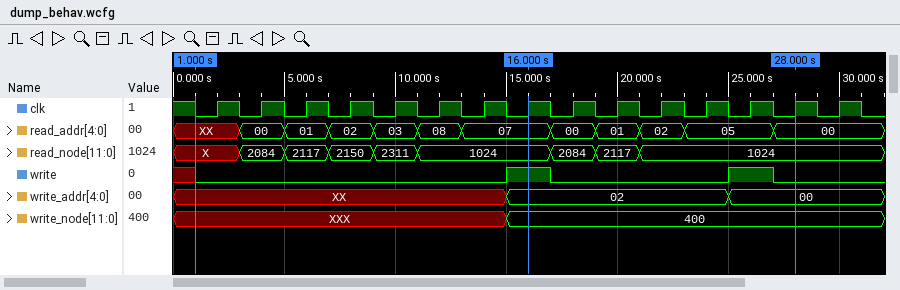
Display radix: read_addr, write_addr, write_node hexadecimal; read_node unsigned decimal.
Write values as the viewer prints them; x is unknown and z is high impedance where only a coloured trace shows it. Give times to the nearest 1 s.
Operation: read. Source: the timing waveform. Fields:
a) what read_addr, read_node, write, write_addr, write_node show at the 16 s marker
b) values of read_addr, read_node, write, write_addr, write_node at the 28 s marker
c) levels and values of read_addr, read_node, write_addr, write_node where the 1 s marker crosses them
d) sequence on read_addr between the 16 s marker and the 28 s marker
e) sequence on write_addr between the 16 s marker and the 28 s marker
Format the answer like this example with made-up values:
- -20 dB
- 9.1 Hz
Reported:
- read_addr=07, read_node=1024, write=1, write_addr=02, write_node=400
- read_addr=00, read_node=1024, write=0, write_addr=00, write_node=400
- read_addr=XX, read_node=X, write_addr=XX, write_node=XXX
- 07, 00, 01, 02, 05, 00
- 02, 00
